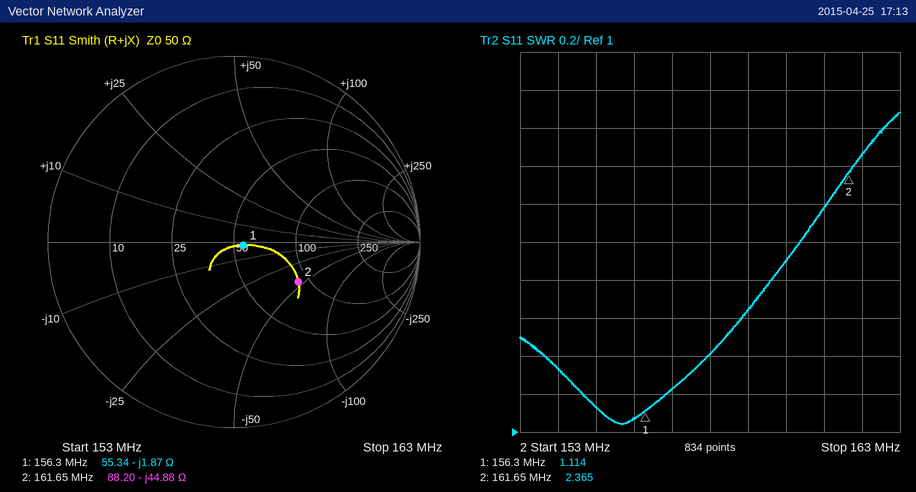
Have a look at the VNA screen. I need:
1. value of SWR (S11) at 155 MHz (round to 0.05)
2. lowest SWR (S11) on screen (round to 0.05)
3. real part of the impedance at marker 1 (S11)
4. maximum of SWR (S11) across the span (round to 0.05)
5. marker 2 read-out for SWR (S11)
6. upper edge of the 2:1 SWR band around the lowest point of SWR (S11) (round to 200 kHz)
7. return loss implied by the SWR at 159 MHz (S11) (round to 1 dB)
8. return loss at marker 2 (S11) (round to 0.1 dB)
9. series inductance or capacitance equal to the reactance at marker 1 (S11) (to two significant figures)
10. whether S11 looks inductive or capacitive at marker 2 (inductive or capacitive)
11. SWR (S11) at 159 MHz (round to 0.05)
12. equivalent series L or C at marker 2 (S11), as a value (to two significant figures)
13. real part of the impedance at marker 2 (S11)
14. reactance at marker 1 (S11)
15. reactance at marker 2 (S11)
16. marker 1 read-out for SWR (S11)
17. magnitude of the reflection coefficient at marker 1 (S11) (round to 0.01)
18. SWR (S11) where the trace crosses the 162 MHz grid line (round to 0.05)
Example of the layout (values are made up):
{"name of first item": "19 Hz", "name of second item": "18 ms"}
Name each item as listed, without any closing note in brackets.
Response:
{"value of SWR (S11) at 155 MHz": "1.15", "lowest SWR (S11) on screen": "1.05", "real part of the impedance at marker 1": "55.34 Ω", "maximum of SWR (S11) across the span": "2.70", "marker 2 read-out for SWR": "2.365", "upper edge of the 2:1 SWR band around the lowest point of SWR (S11)": "160.4 MHz", "return loss implied by the SWR at 159 MHz (S11)": "12 dB", "return loss at marker 2 (S11)": "7.8 dB", "series inductance or capacitance equal to the reactance at marker 1 (S11)": "540 pF", "whether S11 looks inductive or capacitive at marker 2": "capacitive", "SWR (S11) at 159 MHz": "1.65", "equivalent series L or C at marker 2 (S11), as a value": "22 pF", "real part of the impedance at marker 2": "88.20 Ω", "reactance at marker 1": "-1.87 Ω", "reactance at marker 2": "-44.88 Ω", "marker 1 read-out for SWR": "1.114", "magnitude of the reflection coefficient at marker 1 (S11)": "0.05", "SWR (S11) where the trace crosses the 162 MHz grid line": "2.45"}
